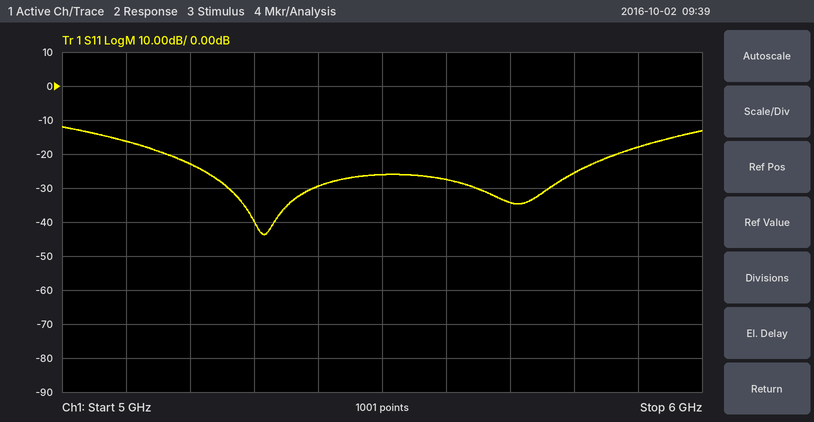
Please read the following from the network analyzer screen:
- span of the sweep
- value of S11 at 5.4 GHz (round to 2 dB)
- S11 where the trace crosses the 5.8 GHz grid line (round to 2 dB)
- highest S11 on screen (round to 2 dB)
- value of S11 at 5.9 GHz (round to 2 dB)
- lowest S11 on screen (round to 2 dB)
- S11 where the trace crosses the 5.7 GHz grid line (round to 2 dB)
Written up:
1 GHz
-30 dB
-26 dB
-12 dB
-18 dB
-44 dB
-34 dB
